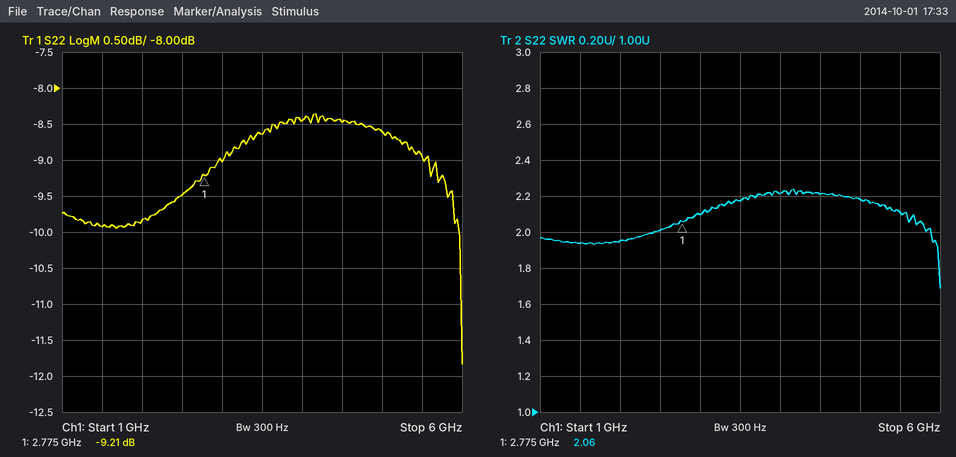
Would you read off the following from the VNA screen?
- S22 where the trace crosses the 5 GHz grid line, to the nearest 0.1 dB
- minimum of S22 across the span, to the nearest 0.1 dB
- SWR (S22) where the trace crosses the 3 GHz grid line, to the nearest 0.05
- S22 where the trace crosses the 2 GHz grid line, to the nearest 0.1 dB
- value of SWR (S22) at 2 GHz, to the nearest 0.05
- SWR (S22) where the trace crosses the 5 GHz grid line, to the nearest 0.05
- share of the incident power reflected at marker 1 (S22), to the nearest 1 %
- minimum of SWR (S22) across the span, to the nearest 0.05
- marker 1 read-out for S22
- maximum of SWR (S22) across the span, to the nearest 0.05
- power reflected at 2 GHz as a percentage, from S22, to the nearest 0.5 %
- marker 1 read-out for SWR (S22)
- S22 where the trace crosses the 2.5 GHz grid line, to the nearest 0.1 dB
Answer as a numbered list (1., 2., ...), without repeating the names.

1. -8.6 dB
2. -11.8 dB
3. 2.10
4. -9.8 dB
5. 1.95
6. 2.20
7. 12 %
8. 1.70
9. -9.21 dB
10. 2.25
11. 10.5 %
12. 2.06
13. -9.5 dB
